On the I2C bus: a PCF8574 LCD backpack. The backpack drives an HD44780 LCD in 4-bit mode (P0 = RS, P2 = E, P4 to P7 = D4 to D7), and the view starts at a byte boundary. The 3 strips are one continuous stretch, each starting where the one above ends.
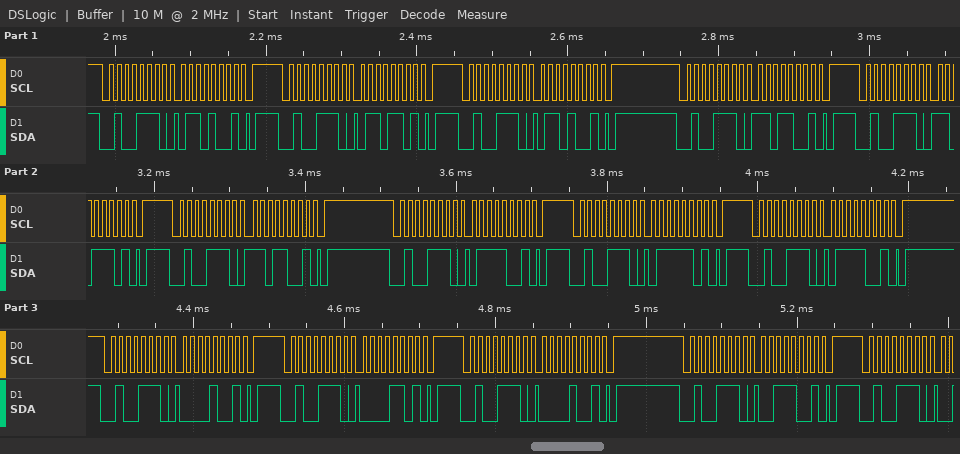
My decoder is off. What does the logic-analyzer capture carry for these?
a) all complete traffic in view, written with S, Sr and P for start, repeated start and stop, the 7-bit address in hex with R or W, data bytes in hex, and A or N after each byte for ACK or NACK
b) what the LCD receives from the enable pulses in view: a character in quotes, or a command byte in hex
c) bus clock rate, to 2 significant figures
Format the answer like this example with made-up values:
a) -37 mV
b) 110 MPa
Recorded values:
a) S 27W A 69 A P S 27W A 6D A P S 27W A 69 A P S 27W A D9 A P S 27W A DD A P S 27W A D9 A P S 27W A 79 A P S 27W A 7D A P S 27W A 79 A P S 27W A 09 A P S 27W A 0D A P S 27W A 09 A P S 27W A 39 A P S 27W A
b) 'm' 'p'
c) 100 kHz
